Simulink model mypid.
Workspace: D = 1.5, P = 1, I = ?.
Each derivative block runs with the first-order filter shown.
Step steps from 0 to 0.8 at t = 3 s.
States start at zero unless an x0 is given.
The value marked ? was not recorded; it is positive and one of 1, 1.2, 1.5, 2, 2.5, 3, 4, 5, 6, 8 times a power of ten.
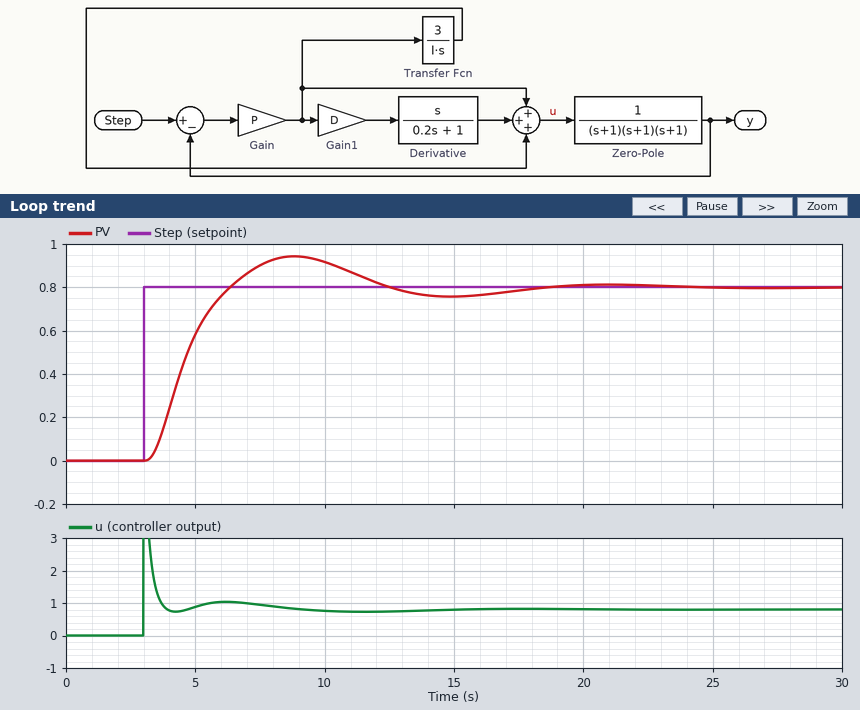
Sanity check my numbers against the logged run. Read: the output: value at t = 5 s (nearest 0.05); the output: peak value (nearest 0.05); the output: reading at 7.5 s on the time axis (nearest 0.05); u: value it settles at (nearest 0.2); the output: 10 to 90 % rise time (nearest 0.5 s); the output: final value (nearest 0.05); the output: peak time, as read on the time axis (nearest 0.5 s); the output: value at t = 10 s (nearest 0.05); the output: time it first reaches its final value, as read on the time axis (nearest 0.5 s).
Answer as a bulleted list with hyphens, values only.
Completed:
- 0.60
- 0.95
- 0.90
- 0.8
- 2.0 s
- 0.80
- 9.0 s
- 0.90
- 6.5 s
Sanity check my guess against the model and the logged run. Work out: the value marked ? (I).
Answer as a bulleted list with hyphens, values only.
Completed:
- 3
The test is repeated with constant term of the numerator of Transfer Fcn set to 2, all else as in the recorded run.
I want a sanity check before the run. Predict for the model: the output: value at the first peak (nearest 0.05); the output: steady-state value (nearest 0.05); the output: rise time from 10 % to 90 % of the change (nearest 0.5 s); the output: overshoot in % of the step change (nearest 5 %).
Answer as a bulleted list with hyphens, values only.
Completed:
- 0.85
- 0.80
- 3.5 s
- 10 %
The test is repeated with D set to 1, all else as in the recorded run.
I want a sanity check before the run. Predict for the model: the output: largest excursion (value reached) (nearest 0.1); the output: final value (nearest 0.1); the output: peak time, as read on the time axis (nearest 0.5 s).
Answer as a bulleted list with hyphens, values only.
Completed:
- 1.0
- 0.8
- 8.0 s
